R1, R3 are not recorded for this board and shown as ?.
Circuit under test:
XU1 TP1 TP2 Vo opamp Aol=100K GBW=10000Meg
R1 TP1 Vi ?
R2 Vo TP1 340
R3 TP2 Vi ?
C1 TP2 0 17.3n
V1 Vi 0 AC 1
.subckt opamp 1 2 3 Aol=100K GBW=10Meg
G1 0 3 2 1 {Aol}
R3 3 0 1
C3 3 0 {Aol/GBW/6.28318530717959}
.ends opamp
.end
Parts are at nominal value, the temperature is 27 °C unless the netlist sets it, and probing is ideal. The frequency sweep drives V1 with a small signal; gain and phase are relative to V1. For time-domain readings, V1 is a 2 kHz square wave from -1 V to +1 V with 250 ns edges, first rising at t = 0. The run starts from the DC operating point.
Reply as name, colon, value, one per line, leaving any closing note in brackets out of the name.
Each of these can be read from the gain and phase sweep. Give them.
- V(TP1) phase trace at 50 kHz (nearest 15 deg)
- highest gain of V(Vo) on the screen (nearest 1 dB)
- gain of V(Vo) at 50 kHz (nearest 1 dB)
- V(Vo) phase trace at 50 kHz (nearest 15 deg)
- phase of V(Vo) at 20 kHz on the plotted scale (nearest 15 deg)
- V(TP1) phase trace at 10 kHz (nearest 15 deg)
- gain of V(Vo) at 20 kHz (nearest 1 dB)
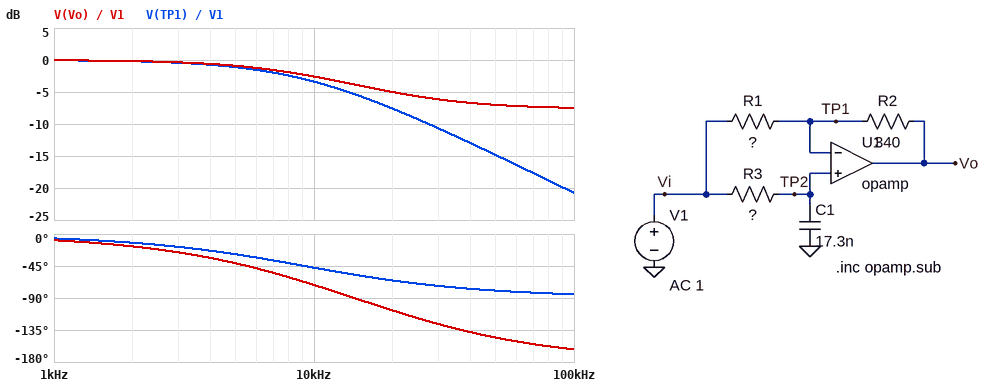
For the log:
V(TP1) phase trace at 50 kHz: -75 deg
highest gain of V(Vo) on the screen: 0 dB
gain of V(Vo) at 50 kHz: -7 dB
V(Vo) phase trace at 50 kHz: -150 deg
phase of V(Vo) at 20 kHz on the plotted scale: -105 deg
V(TP1) phase trace at 10 kHz: -45 deg
gain of V(Vo) at 20 kHz: -5 dB
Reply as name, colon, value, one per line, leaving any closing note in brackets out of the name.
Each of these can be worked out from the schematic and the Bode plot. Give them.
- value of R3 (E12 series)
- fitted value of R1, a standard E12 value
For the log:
value of R3: 1 kΩ
fitted value of R1, a standard E12 value: 820 Ω
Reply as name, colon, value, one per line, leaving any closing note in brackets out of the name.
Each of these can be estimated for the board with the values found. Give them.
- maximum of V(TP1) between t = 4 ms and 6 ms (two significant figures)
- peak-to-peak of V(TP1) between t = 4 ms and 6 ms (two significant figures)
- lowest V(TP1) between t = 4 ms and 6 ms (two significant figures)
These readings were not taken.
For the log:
maximum of V(TP1) between t = 4 ms and 6 ms: 1.0 V
peak-to-peak of V(TP1) between t = 4 ms and 6 ms: 2.0 V
lowest V(TP1) between t = 4 ms and 6 ms: -1.0 V
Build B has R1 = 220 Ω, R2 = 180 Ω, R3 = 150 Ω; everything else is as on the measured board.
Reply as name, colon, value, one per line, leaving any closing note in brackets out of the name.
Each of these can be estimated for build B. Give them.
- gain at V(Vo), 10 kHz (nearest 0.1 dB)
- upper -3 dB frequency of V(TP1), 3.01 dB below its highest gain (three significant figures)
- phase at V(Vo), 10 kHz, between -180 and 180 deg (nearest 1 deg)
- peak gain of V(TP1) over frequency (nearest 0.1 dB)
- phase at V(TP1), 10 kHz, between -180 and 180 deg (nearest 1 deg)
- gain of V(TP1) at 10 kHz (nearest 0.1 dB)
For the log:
gain at V(Vo), 10 kHz: 0 dB
upper -3 dB frequency of V(TP1), 3.01 dB below its highest gain: 61.3 kHz
phase at V(Vo), 10 kHz, between -180 and 180 deg: -17 deg
peak gain of V(TP1) over frequency: 0 dB
phase at V(TP1), 10 kHz, between -180 and 180 deg: -9 deg
gain of V(TP1) at 10 kHz: -0.1 dB
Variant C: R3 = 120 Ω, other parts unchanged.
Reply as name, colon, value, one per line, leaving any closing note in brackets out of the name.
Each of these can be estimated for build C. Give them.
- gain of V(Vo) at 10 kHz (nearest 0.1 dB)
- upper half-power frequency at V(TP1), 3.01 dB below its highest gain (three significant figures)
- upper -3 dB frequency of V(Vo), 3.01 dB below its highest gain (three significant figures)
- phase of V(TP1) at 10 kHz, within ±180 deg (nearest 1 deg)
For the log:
gain of V(Vo) at 10 kHz: -0.1 dB
upper half-power frequency at V(TP1), 3.01 dB below its highest gain: 76.7 kHz
upper -3 dB frequency of V(Vo), 3.01 dB below its highest gain: 94.6 kHz
phase of V(TP1) at 10 kHz, within ±180 deg: -7 deg
